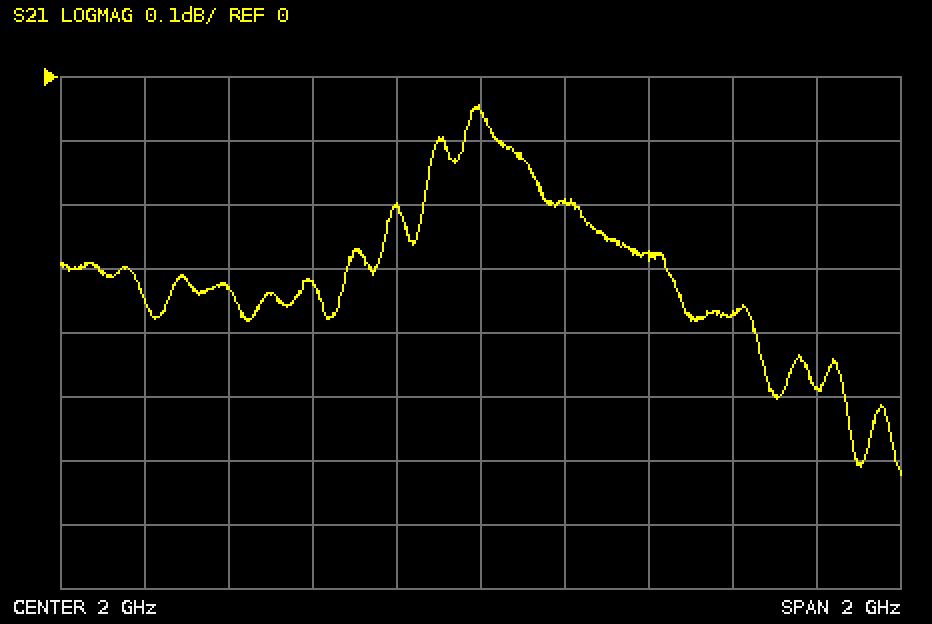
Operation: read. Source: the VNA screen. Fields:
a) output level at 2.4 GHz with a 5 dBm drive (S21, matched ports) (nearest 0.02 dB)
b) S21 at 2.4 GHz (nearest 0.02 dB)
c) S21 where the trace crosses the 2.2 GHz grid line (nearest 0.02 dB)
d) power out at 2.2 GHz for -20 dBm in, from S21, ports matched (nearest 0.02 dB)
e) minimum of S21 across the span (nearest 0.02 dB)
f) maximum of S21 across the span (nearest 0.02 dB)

4.72 dBm
-0.28 dB
-0.20 dB
-20.20 dBm
-0.62 dB
-0.04 dB
